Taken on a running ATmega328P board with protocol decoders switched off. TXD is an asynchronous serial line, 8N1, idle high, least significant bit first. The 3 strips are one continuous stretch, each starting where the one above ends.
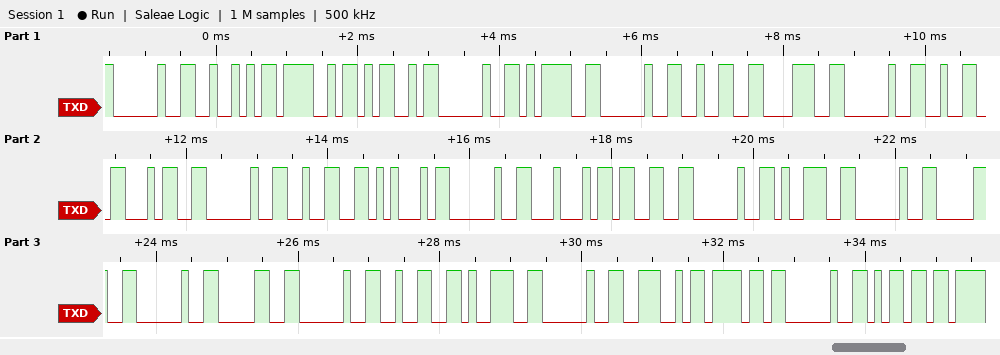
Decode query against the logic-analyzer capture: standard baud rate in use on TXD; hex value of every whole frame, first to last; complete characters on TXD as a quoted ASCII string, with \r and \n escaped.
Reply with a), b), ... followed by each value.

a) 9600 baud
b) 0x20 0x52 0x4F 0x4D 0x20 0x3D 0x20 0x32 0x38 0x20 0x32 0x34 0x20 0x32 0x45 0x20 0x44 0x33 0x20 0x39 0x20 0x30 0x20 0x30 0x20 0x32 0x39 0x20 0x4E 0x6F 0x20 0x6D
c) " ROM = 28 24 2E D3 9 0 0 29 No m"
